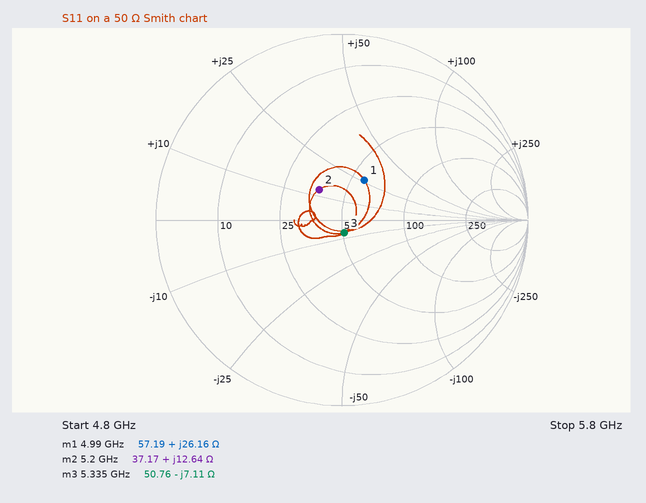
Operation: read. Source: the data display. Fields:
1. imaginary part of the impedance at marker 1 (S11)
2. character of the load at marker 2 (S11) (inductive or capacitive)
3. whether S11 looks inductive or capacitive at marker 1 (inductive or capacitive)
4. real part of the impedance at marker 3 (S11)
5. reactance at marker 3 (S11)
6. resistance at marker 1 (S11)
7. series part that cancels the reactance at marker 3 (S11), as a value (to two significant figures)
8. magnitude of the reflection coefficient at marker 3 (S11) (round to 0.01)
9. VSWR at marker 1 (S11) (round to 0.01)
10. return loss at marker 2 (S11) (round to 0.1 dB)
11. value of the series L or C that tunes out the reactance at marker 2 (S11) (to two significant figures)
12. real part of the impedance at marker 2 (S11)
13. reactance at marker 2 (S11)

+26.16 Ω
inductive
inductive
50.76 Ω
-7.11 Ω
57.19 Ω
210 pH
0.07
1.65
13.8 dB
2.4 pF
37.17 Ω
+12.64 Ω
